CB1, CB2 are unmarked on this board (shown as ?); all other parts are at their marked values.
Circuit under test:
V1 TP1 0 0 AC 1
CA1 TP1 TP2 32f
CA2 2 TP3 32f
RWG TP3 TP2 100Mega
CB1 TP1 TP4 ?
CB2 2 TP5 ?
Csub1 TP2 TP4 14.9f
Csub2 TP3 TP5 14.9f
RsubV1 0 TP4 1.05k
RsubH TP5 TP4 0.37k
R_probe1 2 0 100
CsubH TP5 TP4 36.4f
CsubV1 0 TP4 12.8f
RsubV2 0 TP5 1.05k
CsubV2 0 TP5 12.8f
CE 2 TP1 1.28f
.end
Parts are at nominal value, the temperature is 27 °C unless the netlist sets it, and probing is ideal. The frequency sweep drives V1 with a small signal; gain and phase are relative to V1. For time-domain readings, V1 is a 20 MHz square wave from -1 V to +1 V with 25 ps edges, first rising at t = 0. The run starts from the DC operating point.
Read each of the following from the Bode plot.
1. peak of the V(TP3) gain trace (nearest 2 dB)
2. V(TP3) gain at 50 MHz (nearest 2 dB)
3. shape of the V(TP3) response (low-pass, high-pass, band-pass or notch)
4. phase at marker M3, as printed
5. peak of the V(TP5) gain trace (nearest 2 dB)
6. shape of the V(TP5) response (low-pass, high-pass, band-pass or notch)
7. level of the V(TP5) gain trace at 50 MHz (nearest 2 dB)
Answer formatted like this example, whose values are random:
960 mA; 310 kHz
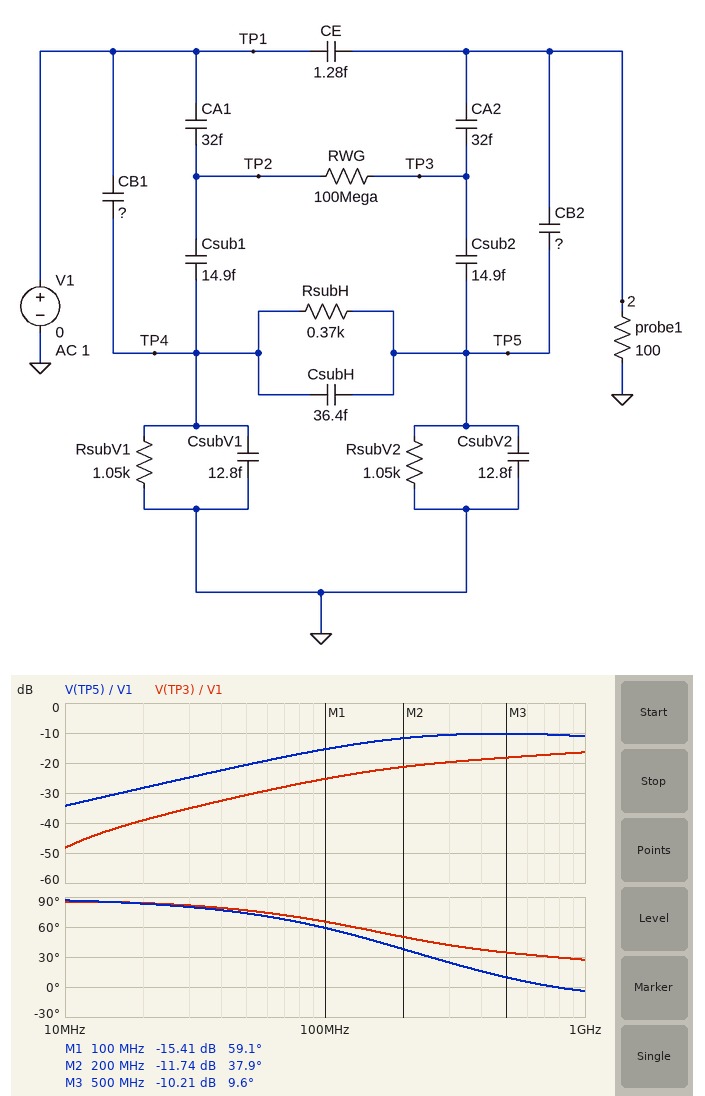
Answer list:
-16 dB; -30 dB; high-pass; 9.6 deg; -10 dB; high-pass; -20 dB
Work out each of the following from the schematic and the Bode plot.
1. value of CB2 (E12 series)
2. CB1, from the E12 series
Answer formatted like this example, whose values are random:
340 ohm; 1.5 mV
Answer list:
820 fF; 680 fF
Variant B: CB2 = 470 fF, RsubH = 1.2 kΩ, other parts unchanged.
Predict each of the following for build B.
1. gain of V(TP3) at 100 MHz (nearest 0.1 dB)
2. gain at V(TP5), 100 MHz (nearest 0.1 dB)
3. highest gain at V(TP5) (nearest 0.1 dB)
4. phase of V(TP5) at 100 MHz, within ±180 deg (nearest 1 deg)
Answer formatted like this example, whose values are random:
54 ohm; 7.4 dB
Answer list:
-27.5 dB; -17.6 dB; -12.0 dB; 61 deg
